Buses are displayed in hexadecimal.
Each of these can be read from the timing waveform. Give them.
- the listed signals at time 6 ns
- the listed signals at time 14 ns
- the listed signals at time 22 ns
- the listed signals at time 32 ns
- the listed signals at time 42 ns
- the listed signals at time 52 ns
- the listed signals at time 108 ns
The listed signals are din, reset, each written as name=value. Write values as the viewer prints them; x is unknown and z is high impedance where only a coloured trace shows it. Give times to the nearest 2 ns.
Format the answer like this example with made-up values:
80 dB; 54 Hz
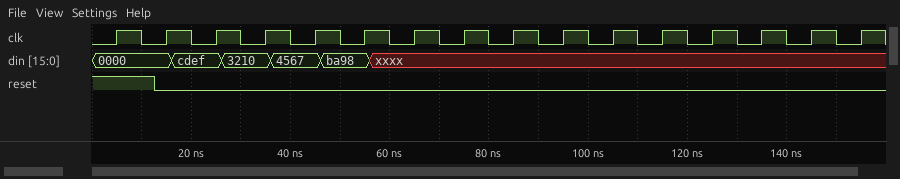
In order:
din=0000, reset=1; din=0000, reset=0; din=cdef, reset=0; din=3210, reset=0; din=4567, reset=0; din=ba98, reset=0; din=xxxx, reset=0
